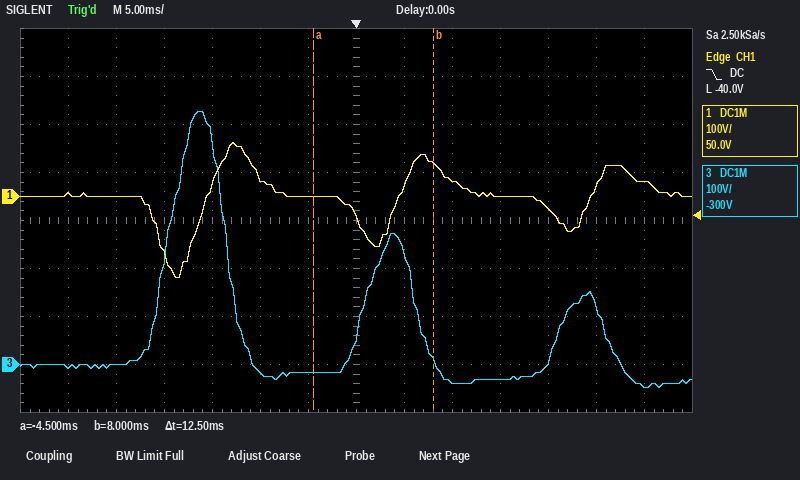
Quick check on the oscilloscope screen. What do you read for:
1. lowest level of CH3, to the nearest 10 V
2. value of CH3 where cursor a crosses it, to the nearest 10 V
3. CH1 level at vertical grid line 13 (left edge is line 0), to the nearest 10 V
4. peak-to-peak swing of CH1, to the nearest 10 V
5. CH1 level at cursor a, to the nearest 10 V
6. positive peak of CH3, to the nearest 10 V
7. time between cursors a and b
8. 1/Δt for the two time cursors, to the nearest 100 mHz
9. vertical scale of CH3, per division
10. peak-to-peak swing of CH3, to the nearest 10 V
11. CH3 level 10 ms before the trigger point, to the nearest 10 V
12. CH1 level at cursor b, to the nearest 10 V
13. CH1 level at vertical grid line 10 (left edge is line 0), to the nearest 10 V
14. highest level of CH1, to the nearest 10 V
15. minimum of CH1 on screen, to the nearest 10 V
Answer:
-50 V
-20 V
30 V
280 V
0 V
530 V
12.5 ms
80.0 Hz
100 V
580 V
-20 V
70 V
0 V
110 V
-170 V
